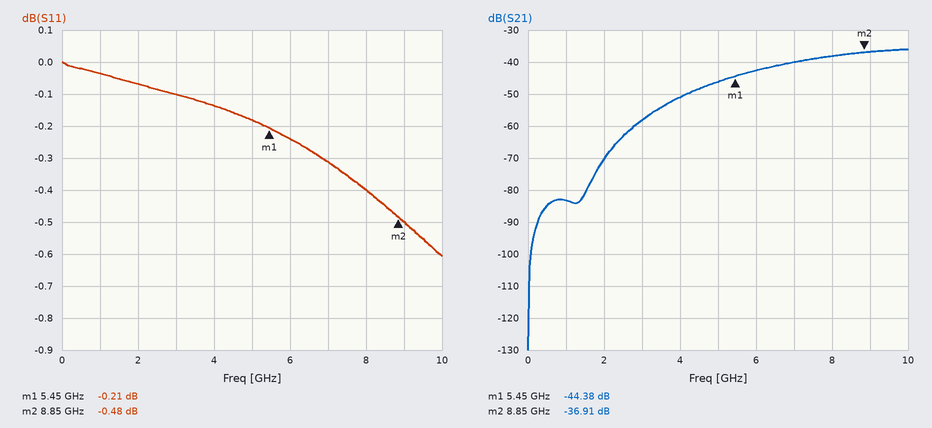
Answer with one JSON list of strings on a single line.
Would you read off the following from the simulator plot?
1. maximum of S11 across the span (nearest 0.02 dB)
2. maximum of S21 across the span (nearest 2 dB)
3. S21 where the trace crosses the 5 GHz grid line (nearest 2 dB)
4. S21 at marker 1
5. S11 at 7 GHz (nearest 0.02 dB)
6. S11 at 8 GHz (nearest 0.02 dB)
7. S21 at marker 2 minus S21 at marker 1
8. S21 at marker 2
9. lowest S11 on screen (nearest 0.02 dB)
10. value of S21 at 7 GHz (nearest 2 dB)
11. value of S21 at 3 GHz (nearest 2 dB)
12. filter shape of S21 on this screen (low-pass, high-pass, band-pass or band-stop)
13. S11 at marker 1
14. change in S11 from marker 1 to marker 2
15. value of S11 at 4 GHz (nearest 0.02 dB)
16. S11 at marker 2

["0.00 dB", "-36 dB", "-46 dB", "-44.38 dB", "-0.32 dB", "-0.40 dB", "7.47 dB", "-36.91 dB", "-0.60 dB", "-40 dB", "-58 dB", "high-pass", "-0.21 dB", "-0.27 dB", "-0.14 dB", "-0.48 dB"]
